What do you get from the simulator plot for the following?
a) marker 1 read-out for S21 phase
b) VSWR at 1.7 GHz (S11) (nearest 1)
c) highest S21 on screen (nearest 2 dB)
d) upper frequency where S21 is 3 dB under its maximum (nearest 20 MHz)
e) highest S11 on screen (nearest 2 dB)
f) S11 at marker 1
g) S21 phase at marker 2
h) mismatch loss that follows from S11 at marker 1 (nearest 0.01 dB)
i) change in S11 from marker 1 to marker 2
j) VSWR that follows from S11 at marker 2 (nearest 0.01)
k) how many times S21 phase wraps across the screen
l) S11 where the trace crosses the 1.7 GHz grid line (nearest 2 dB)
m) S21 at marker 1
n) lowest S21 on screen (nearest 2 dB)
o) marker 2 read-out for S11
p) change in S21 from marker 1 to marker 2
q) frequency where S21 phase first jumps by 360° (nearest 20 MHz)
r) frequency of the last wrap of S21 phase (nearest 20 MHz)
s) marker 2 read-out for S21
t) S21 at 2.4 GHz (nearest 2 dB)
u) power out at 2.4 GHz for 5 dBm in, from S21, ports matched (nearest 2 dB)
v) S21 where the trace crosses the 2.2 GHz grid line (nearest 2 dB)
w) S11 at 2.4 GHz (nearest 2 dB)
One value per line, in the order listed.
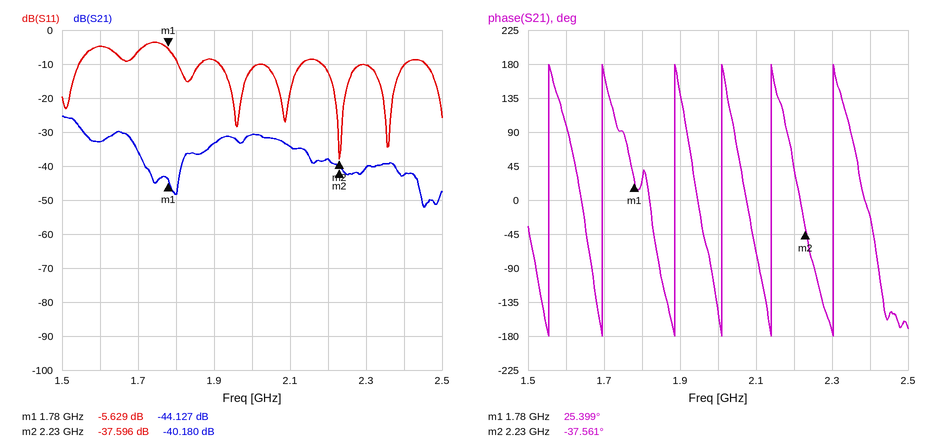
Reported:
25.399°
3
-26 dB
1.54 GHz
-4 dB
-5.629 dB
-37.561°
1.39 dB
-31.967 dB
1.03
6
-6 dB
-44.127 dB
-52 dB
-37.596 dB
3.947 dB
1.56 GHz
2.30 GHz
-40.180 dB
-42 dB
-38 dBm
-38 dB
-10 dB
